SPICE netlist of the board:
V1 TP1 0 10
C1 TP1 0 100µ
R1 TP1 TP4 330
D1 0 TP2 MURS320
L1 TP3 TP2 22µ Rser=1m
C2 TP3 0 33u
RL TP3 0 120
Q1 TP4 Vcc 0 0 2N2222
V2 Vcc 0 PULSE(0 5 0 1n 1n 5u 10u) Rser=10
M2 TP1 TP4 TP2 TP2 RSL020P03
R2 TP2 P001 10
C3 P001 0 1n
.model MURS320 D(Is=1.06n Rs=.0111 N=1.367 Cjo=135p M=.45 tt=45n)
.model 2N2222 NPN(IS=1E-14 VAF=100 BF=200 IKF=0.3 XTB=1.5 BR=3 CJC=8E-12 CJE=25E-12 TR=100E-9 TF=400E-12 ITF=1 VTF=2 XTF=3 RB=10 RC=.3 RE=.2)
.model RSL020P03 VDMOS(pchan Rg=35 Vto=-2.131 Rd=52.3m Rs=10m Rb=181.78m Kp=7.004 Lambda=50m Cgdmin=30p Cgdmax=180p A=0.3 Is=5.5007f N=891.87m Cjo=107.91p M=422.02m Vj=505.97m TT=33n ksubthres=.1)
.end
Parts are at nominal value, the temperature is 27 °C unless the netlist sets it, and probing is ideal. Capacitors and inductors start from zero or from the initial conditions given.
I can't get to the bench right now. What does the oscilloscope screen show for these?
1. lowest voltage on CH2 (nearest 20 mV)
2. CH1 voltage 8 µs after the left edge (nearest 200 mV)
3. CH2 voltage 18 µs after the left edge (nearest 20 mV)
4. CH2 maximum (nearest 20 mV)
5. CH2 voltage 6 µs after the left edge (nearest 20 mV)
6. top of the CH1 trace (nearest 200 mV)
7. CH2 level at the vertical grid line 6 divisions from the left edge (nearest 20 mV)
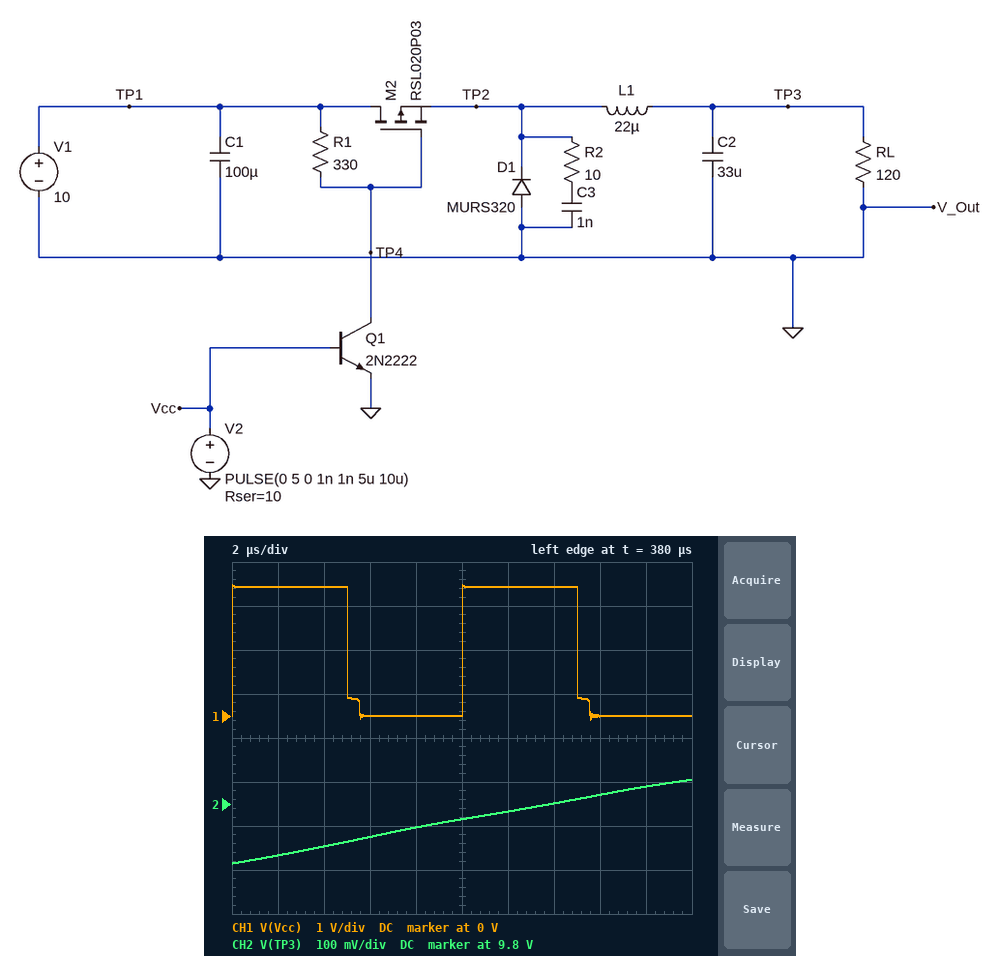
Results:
9.66 V
0 V
9.84 V
9.86 V
9.72 V
3.0 V
9.78 V
